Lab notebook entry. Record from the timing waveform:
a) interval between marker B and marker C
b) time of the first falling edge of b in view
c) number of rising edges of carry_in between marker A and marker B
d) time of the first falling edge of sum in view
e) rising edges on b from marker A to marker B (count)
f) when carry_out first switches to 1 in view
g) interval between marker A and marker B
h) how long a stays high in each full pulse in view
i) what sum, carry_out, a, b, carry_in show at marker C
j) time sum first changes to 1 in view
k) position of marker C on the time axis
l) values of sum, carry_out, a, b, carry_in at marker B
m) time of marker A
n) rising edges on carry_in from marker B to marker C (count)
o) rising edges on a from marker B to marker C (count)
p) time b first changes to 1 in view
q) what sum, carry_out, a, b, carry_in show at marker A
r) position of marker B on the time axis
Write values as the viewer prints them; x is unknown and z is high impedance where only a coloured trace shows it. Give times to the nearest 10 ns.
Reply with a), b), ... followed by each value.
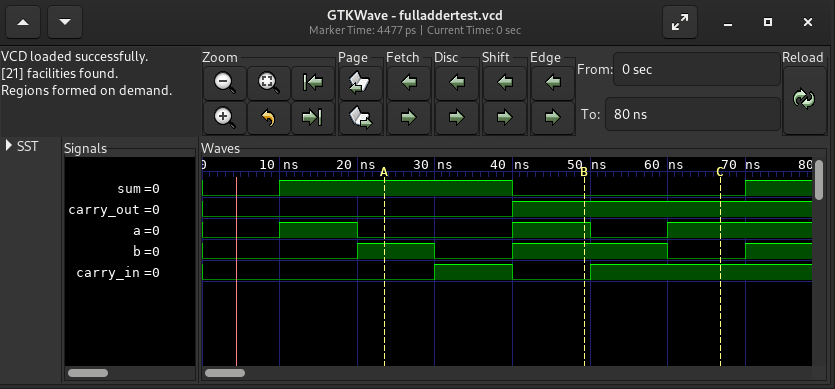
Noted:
a) 20 ns
b) 30 ns
c) 1
d) 40 ns
e) 1
f) 40 ns
g) 30 ns
h) 10 ns, 10 ns
i) sum=0, carry_out=1, a=1, b=0, carry_in=1
j) 10 ns
k) 70 ns
l) sum=0, carry_out=1, a=1, b=1, carry_in=0
m) 20 ns
n) 1
o) 1
p) 20 ns
q) sum=1, carry_out=0, a=0, b=1, carry_in=0
r) 50 ns
